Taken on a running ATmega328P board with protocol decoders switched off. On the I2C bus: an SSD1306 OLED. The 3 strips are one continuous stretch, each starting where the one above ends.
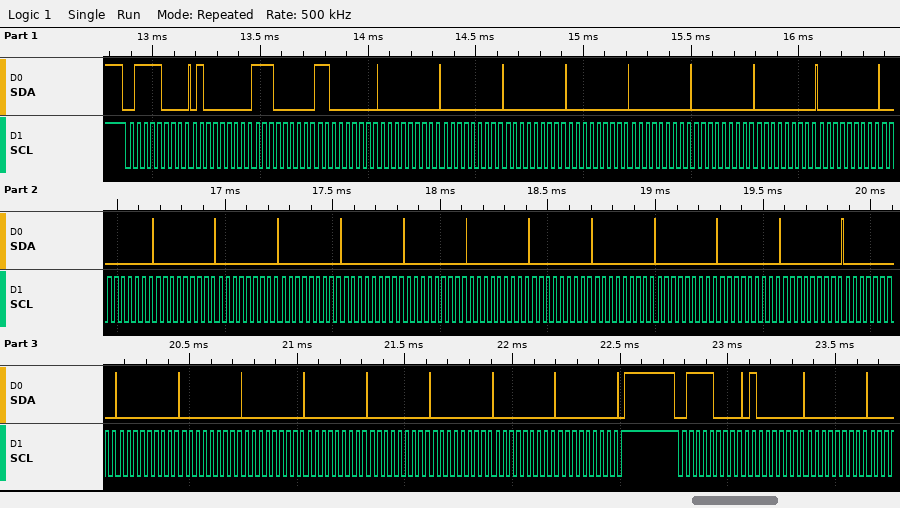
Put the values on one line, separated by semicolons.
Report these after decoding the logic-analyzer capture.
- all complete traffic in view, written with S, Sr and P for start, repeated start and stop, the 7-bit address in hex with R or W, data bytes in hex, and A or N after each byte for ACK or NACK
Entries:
S 3CW A 40 A E0 A C0 A 00 A 00 A 00 A 00 A 00 A 00 A 00 A 00 A 00 A 00 A 00 A 00 A 00 A 00 A 00 A 00 A 00 A 00 A 00 A 00 A 00 A 00 A 00 A 00 A 00 A 00 A 00 A 00 A 00 A P S 3CW A 40 A 00 A
